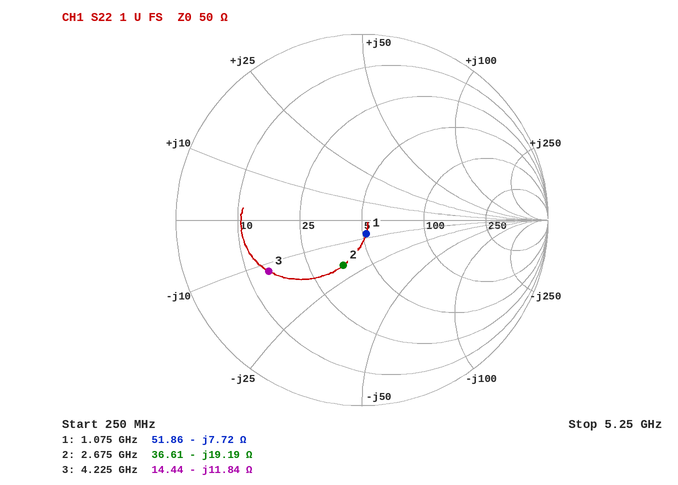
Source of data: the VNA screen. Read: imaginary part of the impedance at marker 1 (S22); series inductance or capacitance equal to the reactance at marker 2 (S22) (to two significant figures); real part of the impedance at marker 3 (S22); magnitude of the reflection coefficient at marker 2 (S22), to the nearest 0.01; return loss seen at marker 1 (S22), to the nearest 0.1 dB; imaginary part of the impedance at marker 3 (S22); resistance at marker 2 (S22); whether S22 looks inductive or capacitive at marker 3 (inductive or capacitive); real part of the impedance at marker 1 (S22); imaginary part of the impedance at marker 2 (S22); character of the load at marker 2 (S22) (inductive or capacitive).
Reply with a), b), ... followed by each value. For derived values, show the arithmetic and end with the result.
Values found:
a) -7.72 Ω
b) C = 1/(2π × 2.675 GHz × 19.19 Ω) ≈ 3.1 pF
c) 14.44 Ω
d) 0.26
e) 22.2 dB
f) -11.84 Ω
g) 36.61 Ω
h) capacitive
i) 51.86 Ω
j) -19.19 Ω
k) capacitive
